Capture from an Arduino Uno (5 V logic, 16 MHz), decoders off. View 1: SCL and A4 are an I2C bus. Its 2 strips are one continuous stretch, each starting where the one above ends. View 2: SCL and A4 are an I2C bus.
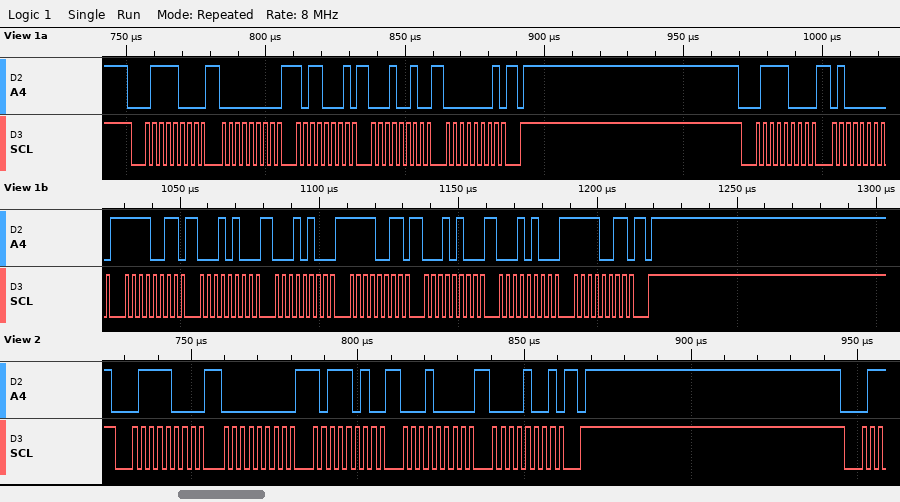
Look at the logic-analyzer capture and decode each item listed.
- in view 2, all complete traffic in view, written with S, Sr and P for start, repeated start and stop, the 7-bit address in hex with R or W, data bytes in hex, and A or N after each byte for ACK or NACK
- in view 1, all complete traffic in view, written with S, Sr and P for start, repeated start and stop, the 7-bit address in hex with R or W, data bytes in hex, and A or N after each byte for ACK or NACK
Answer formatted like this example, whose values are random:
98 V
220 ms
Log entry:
S 3CW A 00 A BA A 10 A 09 A P
S 3CW A 00 A B1 A 12 A 01 A P S 3CW A 40 A F3 A 14 A 14 A F3 A 14 A 14 A F3 A P
